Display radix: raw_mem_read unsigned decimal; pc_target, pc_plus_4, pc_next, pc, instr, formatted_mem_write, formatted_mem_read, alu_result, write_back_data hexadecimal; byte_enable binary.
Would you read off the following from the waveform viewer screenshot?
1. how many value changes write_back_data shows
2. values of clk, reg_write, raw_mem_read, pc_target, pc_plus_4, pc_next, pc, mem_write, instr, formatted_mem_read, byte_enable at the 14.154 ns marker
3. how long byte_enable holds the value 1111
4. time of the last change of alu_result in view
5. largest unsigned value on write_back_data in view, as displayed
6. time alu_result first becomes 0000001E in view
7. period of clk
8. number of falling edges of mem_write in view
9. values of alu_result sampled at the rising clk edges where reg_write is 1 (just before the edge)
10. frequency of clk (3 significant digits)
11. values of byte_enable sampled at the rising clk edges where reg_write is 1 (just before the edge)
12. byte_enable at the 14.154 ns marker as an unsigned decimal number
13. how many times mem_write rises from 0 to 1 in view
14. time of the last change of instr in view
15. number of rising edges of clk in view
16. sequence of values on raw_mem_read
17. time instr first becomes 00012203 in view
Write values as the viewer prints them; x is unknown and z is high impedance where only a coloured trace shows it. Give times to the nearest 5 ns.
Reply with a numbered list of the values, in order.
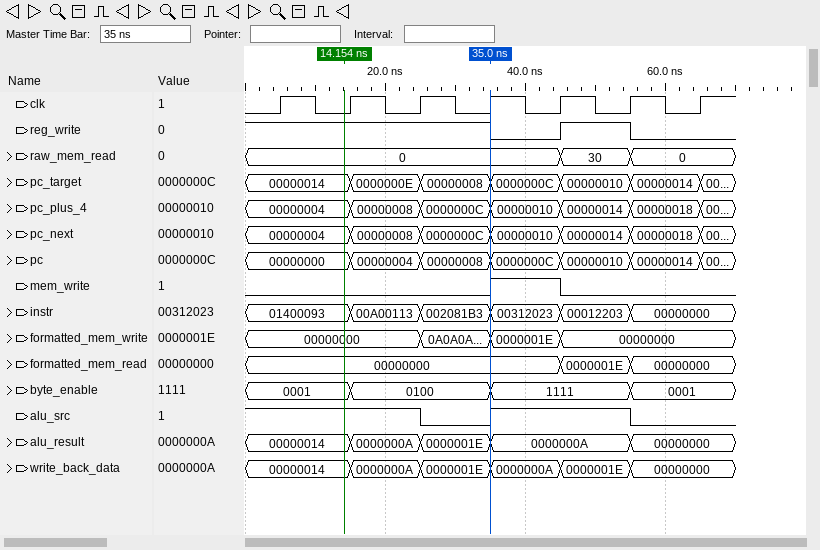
1. 5
2. clk=0, reg_write=1, raw_mem_read=0, pc_target=00000014, pc_plus_4=00000004, pc_next=00000004, pc=00000000, mem_write=0, instr=01400093, formatted_mem_read=00000000, byte_enable=0001
3. 20 ns
4. 55 ns
5. 0000001E
6. 25 ns
7. 10 ns
8. 1
9. 00000014, 00000014, 0000000A, 0000001E, 0000000A
10. 100 MHz
11. 0001, 0001, 0100, 0100, 1111
12. 1
13. 1
14. 55 ns
15. 7
16. 0, 30, 0
17. 45 ns
